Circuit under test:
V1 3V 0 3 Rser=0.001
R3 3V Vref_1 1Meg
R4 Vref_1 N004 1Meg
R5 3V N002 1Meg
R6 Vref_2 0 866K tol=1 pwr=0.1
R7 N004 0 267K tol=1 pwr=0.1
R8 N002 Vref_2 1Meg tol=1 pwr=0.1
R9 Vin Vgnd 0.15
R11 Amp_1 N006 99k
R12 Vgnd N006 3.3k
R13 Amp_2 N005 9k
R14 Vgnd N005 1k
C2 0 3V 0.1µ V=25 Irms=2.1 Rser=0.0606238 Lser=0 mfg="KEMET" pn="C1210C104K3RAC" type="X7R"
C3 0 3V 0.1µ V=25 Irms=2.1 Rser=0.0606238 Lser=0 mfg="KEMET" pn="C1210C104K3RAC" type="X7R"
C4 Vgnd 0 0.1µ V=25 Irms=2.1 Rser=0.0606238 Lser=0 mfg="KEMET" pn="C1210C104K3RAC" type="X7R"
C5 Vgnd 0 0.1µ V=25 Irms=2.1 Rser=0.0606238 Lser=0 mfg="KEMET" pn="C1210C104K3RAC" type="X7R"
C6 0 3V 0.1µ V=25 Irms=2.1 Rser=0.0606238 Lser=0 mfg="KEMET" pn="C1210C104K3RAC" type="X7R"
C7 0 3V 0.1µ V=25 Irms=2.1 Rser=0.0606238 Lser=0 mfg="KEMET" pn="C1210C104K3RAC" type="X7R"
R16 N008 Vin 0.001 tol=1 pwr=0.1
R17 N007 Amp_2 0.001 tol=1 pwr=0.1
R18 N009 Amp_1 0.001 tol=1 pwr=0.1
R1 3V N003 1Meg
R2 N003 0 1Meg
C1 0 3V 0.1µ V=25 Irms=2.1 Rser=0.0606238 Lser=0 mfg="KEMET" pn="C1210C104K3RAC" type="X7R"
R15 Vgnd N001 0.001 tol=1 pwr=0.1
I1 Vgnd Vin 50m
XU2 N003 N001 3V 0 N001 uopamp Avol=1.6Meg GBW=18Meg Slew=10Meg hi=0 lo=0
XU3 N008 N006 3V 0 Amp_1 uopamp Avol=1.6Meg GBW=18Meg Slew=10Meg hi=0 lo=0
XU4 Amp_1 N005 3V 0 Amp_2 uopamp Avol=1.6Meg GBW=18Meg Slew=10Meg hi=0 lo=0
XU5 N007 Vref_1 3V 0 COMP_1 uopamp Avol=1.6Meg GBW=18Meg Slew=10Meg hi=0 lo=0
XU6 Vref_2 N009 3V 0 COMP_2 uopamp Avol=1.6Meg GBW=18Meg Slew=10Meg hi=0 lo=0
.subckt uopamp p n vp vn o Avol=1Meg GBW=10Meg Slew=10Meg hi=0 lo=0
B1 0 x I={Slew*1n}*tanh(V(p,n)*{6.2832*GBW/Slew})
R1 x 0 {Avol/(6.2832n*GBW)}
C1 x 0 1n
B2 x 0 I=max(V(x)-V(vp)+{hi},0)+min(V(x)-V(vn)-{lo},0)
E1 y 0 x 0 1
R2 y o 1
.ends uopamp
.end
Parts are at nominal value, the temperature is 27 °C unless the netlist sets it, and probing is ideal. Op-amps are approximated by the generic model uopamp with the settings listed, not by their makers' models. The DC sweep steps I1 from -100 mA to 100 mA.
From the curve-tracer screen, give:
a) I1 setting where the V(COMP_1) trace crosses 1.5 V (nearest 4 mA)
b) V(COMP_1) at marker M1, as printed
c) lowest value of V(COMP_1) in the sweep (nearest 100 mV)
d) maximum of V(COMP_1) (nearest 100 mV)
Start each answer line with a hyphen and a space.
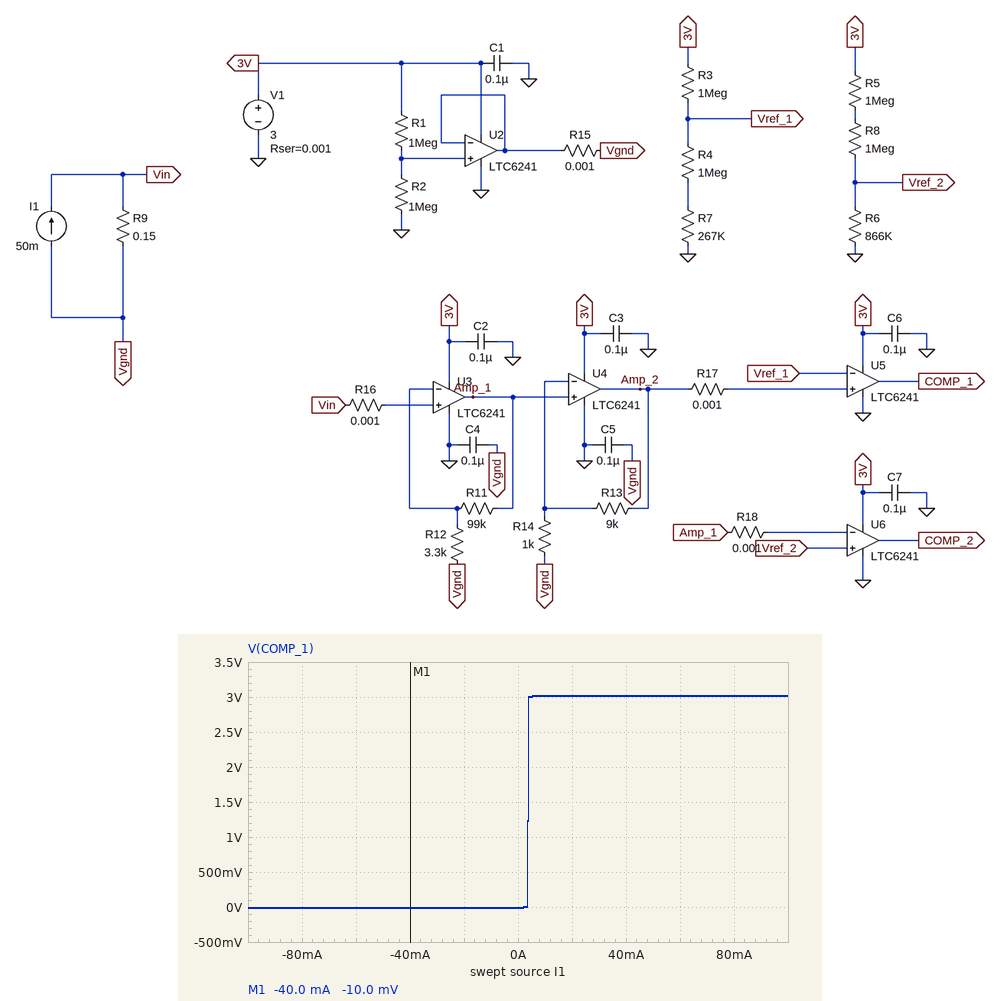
- 4 mA
- -10.0 mV
- 0 V
- 3.0 V
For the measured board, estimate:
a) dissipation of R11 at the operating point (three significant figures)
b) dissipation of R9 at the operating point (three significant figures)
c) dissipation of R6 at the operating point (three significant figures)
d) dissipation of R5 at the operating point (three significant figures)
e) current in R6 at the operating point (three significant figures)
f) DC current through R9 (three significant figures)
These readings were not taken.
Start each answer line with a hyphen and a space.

- 511 nW
- 375 µW
- 949 nW
- 1.10 µW
- 1.05 µA
- 50.0 mA
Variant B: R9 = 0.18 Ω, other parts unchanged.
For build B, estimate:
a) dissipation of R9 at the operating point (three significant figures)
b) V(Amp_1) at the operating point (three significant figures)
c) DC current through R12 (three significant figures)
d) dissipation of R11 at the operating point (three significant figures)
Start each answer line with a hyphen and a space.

- 450 µW
- 1.78 V
- 2.73 µA
- 736 nW
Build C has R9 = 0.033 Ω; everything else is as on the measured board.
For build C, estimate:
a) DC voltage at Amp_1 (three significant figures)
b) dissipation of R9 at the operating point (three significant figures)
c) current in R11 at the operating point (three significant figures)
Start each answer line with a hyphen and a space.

- 1.55 V
- 82.5 µW
- 500 nA
